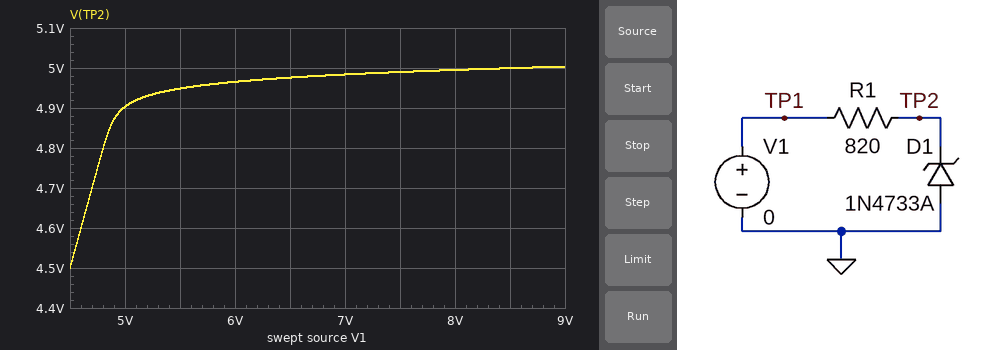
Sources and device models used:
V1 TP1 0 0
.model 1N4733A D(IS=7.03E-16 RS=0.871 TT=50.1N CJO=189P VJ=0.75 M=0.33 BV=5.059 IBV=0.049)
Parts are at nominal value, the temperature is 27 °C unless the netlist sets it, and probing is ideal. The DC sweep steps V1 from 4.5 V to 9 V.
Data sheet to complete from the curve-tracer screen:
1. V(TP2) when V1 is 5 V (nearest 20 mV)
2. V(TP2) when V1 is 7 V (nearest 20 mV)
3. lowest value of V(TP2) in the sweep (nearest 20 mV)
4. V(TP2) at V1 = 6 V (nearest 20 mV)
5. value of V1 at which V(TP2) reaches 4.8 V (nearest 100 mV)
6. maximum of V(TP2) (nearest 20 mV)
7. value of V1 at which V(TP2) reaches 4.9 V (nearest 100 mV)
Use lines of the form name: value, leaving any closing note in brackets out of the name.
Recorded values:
V(TP2) when V1 is 5 V: 4.90 V
V(TP2) when V1 is 7 V: 4.98 V
lowest value of V(TP2) in the sweep: 4.50 V
V(TP2) at V1 = 6 V: 4.96 V
value of V1 at which V(TP2) reaches 4.8 V: 4.8 V
maximum of V(TP2): 5.00 V
value of V1 at which V(TP2) reaches 4.9 V: 5.0 V
